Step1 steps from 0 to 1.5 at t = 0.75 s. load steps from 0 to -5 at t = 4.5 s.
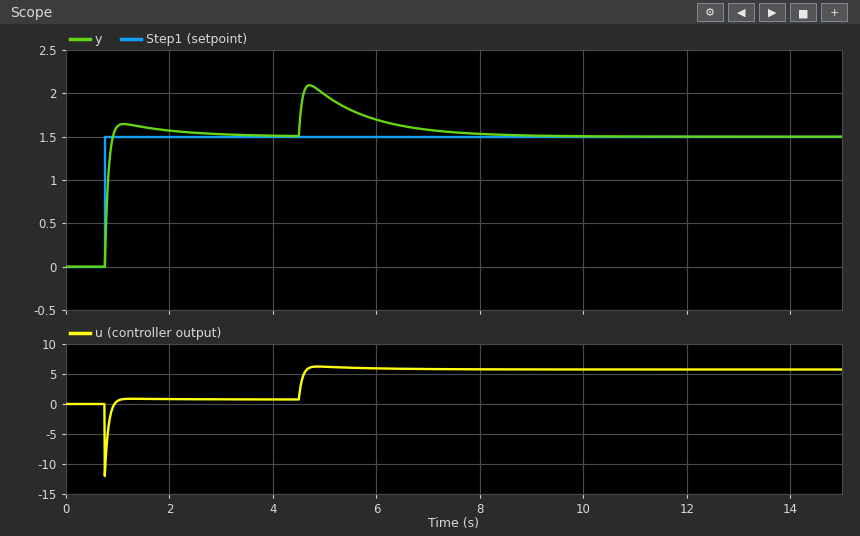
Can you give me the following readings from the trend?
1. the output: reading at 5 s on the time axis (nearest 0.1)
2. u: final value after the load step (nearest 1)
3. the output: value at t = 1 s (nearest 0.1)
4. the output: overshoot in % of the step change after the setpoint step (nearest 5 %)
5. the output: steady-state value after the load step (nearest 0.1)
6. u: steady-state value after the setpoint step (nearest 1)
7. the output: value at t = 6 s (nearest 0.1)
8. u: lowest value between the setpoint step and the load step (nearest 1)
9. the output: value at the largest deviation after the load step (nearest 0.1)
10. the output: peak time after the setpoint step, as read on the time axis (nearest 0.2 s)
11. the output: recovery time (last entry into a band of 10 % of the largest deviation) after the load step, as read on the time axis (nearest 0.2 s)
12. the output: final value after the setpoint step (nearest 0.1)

2.0
6
1.6
10 %
1.5
1
1.7
-12
2.1
1.2 s
7.4 s
1.5
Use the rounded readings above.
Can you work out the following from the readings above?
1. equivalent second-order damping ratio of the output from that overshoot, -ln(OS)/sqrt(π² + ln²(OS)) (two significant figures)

0.59
